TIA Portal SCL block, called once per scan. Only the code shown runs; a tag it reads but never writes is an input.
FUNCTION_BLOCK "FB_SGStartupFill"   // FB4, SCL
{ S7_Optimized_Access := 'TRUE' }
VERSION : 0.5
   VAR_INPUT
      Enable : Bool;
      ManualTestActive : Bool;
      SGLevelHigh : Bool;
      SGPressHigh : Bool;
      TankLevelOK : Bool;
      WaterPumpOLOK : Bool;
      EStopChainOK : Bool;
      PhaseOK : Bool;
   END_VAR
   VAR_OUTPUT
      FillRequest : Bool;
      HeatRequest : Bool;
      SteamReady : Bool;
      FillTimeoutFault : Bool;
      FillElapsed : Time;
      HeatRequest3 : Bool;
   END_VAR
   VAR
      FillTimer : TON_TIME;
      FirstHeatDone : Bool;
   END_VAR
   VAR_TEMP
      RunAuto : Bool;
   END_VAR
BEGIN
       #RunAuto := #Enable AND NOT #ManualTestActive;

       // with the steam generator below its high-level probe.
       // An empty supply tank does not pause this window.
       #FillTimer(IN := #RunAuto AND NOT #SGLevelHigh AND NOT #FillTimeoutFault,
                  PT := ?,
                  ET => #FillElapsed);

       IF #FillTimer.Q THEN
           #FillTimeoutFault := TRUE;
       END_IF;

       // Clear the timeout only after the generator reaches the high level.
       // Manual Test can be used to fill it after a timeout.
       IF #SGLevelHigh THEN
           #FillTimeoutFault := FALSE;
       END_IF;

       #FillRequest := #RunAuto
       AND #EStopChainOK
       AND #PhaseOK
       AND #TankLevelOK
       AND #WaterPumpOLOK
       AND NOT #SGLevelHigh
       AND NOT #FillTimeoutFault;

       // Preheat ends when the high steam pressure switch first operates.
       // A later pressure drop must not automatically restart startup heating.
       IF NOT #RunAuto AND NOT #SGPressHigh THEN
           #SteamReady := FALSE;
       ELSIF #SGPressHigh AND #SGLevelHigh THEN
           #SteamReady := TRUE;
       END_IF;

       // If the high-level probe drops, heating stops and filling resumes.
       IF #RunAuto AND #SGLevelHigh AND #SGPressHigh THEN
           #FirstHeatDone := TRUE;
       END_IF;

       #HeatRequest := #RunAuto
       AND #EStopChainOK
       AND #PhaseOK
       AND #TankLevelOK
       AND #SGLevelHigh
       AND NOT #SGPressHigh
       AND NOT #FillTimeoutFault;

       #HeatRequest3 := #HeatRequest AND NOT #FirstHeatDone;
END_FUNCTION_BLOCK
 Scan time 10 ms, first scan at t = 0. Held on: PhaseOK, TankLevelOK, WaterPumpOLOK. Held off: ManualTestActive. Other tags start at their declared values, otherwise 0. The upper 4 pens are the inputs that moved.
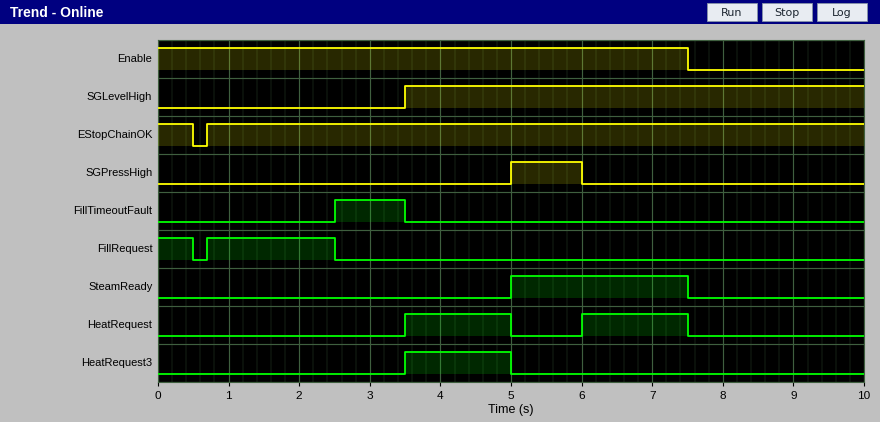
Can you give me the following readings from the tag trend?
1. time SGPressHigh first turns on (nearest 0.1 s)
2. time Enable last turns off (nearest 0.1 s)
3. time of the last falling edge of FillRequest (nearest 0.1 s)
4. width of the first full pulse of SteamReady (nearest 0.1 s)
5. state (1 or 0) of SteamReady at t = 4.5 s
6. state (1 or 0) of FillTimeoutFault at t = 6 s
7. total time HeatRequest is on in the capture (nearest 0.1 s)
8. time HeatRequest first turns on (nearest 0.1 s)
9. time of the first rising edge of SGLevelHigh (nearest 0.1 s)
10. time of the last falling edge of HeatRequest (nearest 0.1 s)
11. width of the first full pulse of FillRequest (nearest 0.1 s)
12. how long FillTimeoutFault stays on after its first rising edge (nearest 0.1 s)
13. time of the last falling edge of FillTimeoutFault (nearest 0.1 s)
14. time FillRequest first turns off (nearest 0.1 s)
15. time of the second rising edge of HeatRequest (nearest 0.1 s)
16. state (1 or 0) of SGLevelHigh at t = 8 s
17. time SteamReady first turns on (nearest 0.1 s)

5.0 s
7.5 s
2.5 s
2.5 s
0
0
3.0 s
3.5 s
3.5 s
7.5 s
1.8 s
1.0 s
3.5 s
0.5 s
6.0 s
1
5.0 s
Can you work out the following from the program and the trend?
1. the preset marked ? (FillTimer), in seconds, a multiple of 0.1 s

2.5 s
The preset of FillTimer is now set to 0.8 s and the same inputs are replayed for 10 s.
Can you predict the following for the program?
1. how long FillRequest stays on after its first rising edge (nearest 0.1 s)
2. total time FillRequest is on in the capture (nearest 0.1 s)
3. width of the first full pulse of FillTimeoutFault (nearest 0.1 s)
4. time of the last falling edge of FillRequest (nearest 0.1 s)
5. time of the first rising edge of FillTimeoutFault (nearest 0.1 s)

0.1 s
0.6 s
2.7 s
0.8 s
0.8 s
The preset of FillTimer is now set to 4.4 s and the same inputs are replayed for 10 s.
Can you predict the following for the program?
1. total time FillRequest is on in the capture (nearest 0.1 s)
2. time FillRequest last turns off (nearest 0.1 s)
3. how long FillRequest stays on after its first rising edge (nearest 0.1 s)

3.3 s
3.5 s
2.8 s
